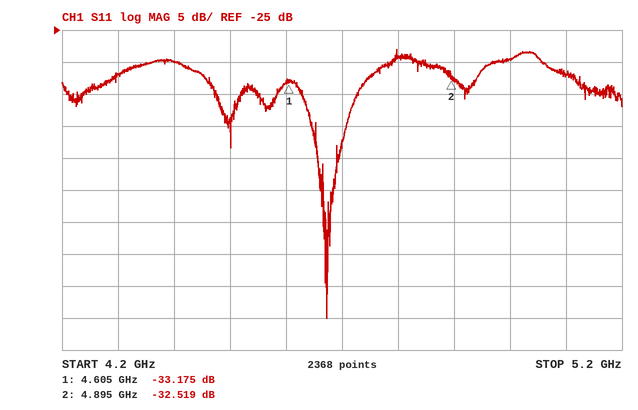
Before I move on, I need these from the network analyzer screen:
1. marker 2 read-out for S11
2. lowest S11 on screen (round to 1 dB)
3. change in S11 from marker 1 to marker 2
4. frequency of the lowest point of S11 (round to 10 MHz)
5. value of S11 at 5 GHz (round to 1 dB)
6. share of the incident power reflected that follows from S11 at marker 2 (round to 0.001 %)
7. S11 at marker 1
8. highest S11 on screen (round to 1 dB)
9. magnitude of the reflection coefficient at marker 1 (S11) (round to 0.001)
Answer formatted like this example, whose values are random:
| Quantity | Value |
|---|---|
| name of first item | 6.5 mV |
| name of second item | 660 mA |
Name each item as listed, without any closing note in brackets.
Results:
| Quantity | Value |
|---|---|
| marker 2 read-out for S11 | -32.519 dB |
| lowest S11 on screen | -70 dB |
| change in S11 from marker 1 to marker 2 | 0.656 dB |
| frequency of the lowest point of S11 | 4.67 GHz |
| value of S11 at 5 GHz | -30 dB |
| share of the incident power reflected that follows from S11 at marker 2 | 0.056 % |
| S11 at marker 1 | -33.175 dB |
| highest S11 on screen | -28 dB |
| magnitude of the reflection coefficient at marker 1 (S11) | 0.022 |
